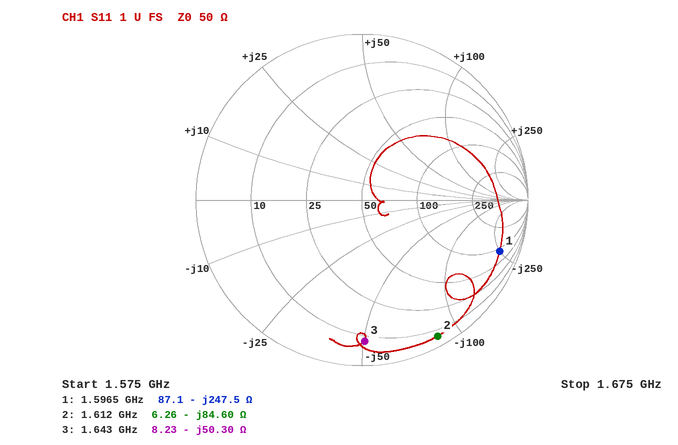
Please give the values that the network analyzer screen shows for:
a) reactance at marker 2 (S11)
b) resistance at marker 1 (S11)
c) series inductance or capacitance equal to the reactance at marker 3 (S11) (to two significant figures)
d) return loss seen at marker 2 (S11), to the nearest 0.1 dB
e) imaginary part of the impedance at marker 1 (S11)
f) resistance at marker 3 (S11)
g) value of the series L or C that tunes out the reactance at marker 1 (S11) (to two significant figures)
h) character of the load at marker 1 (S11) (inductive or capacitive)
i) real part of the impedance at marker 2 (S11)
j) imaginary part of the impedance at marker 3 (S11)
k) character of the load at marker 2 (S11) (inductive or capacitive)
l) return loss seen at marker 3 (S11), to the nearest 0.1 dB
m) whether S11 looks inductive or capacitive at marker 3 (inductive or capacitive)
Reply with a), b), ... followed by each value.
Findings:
a) -84.60 Ω
b) 87.1 Ω
c) 1.9 pF
d) 0.6 dB
e) -247.5 Ω
f) 8.23 Ω
g) 25 nH
h) capacitive
i) 6.26 Ω
j) -50.30 Ω
k) capacitive
l) 1.4 dB
m) capacitive
